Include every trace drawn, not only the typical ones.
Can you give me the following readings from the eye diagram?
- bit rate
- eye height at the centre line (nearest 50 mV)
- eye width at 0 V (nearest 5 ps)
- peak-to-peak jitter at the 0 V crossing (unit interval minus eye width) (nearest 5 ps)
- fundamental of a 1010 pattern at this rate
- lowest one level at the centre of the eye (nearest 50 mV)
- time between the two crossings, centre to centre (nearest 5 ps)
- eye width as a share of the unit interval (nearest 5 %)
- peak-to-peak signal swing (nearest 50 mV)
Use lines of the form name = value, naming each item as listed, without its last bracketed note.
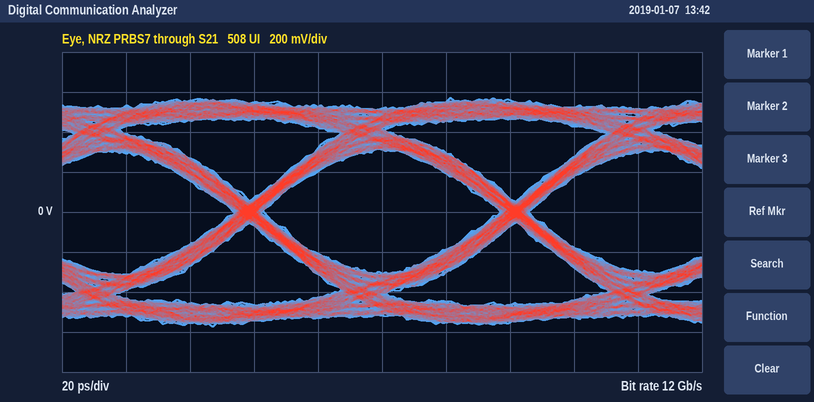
bit rate = 12 Gb/s
eye height at the centre line = 600 mV
eye width at 0 V = 75 ps
peak-to-peak jitter at the 0 V crossing (unit interval minus eye width) = 10 ps
fundamental of a 1010 pattern at this rate = 6 GHz
lowest one level at the centre of the eye = 300 mV
time between the two crossings, centre to centre = 85 ps
eye width as a share of the unit interval = 90 %
peak-to-peak signal swing = 1.15 V
